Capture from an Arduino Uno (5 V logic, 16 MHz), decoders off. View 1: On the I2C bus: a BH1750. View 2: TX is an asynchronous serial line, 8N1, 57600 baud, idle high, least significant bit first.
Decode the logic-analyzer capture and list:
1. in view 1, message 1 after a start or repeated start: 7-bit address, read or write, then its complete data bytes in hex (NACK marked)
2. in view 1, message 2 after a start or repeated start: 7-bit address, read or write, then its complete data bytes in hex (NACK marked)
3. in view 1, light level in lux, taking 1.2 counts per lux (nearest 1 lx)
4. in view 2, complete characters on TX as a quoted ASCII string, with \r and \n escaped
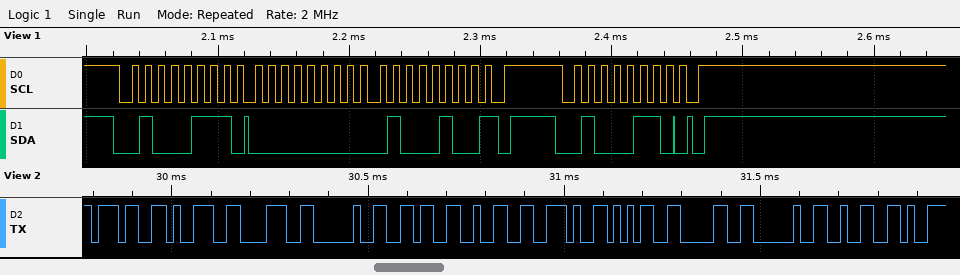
0x23 read: 00 44 NACK
0x23 write
57 lx
"798 62.50 2"
